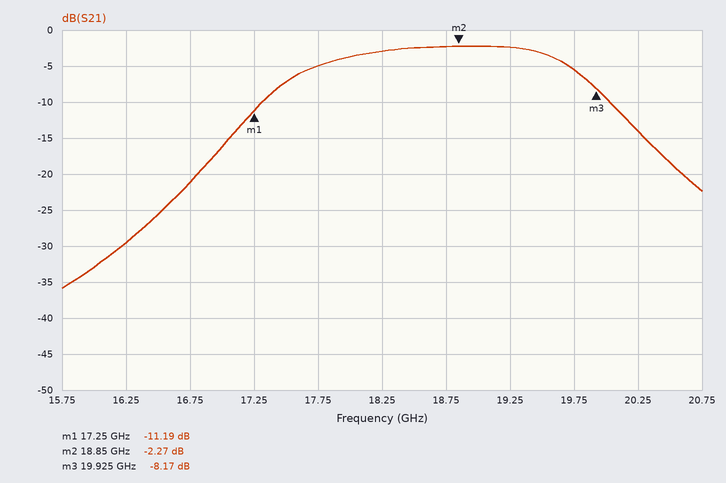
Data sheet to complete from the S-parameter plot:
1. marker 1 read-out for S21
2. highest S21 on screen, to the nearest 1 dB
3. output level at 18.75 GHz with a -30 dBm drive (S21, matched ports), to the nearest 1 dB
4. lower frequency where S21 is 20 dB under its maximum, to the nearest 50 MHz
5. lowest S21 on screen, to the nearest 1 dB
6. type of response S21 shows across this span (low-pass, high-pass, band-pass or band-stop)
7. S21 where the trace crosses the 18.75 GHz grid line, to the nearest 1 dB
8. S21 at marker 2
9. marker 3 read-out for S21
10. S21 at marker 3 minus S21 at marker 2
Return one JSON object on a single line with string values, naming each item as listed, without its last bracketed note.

{"marker 1 read-out for S21": "-11.19 dB", "highest S21 on screen, to the nearest 1 dB": "-2 dB", "output level at 18.75 GHz with a -30 dBm drive (S21, matched ports), to the nearest 1 dB": "-32 dBm", "lower frequency where S21 is 20 dB under its maximum, to the nearest 50 MHz": "16.70 GHz", "lowest S21 on screen, to the nearest 1 dB": "-36 dB", "type of response S21 shows across this span": "band-pass", "S21 where the trace crosses the 18.75 GHz grid line, to the nearest 1 dB": "-2 dB", "S21 at marker 2": "-2.27 dB", "marker 3 read-out for S21": "-8.17 dB", "S21 at marker 3 minus S21 at marker 2": "-5.90 dB"}
